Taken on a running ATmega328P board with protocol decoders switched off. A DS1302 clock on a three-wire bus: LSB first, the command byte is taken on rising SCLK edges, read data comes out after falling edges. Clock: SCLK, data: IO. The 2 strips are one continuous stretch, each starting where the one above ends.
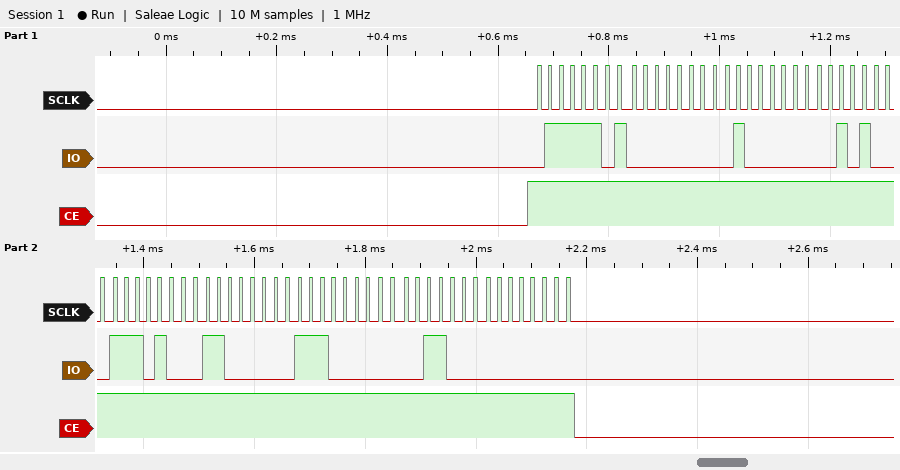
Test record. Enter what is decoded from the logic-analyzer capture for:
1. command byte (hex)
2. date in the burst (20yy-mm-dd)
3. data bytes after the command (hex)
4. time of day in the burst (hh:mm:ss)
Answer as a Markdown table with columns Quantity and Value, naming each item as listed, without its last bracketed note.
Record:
| Quantity | Value |
|---|---|
| command byte | 0xBE |
| date in the burst | 2018-03-17 |
| data bytes after the command | 00 02 14 17 03 07 18 00 |
| time of day in the burst | 14:02:00 |
